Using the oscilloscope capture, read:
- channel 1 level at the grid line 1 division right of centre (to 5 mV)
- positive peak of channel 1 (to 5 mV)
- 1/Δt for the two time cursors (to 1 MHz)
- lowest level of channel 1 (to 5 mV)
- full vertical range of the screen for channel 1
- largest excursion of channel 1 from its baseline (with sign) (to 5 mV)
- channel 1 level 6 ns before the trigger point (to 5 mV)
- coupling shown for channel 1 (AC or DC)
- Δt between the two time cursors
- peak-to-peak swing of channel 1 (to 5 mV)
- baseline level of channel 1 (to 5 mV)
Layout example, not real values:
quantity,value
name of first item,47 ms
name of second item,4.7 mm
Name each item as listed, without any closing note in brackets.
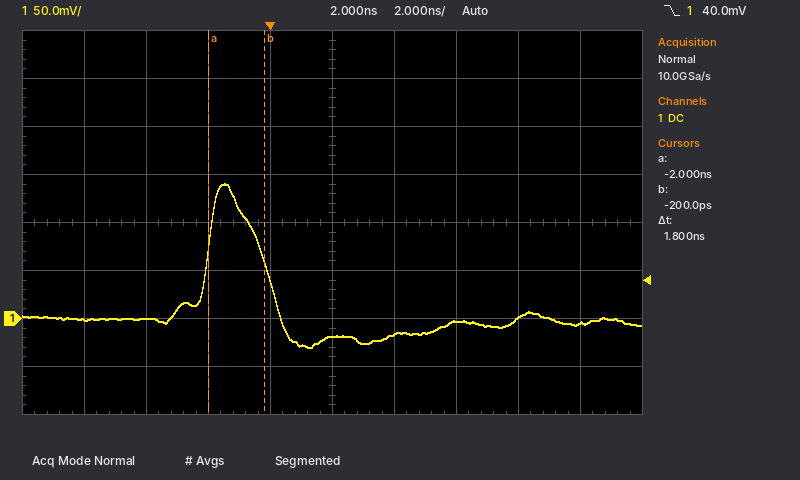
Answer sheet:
quantity,value
channel 1 level at the grid line 1 division right of centre,-15 mV
positive peak of channel 1,140 mV
1/Δt for the two time cursors,556 MHz
lowest level of channel 1,-30 mV
full vertical range of the screen for channel 1,400 mV
largest excursion of channel 1 from its baseline (with sign),+140 mV
channel 1 level 6 ns before the trigger point,0 mV
coupling shown for channel 1,DC
Δt between the two time cursors,1.8 ns
peak-to-peak swing of channel 1,170 mV
baseline level of channel 1,0 mV
